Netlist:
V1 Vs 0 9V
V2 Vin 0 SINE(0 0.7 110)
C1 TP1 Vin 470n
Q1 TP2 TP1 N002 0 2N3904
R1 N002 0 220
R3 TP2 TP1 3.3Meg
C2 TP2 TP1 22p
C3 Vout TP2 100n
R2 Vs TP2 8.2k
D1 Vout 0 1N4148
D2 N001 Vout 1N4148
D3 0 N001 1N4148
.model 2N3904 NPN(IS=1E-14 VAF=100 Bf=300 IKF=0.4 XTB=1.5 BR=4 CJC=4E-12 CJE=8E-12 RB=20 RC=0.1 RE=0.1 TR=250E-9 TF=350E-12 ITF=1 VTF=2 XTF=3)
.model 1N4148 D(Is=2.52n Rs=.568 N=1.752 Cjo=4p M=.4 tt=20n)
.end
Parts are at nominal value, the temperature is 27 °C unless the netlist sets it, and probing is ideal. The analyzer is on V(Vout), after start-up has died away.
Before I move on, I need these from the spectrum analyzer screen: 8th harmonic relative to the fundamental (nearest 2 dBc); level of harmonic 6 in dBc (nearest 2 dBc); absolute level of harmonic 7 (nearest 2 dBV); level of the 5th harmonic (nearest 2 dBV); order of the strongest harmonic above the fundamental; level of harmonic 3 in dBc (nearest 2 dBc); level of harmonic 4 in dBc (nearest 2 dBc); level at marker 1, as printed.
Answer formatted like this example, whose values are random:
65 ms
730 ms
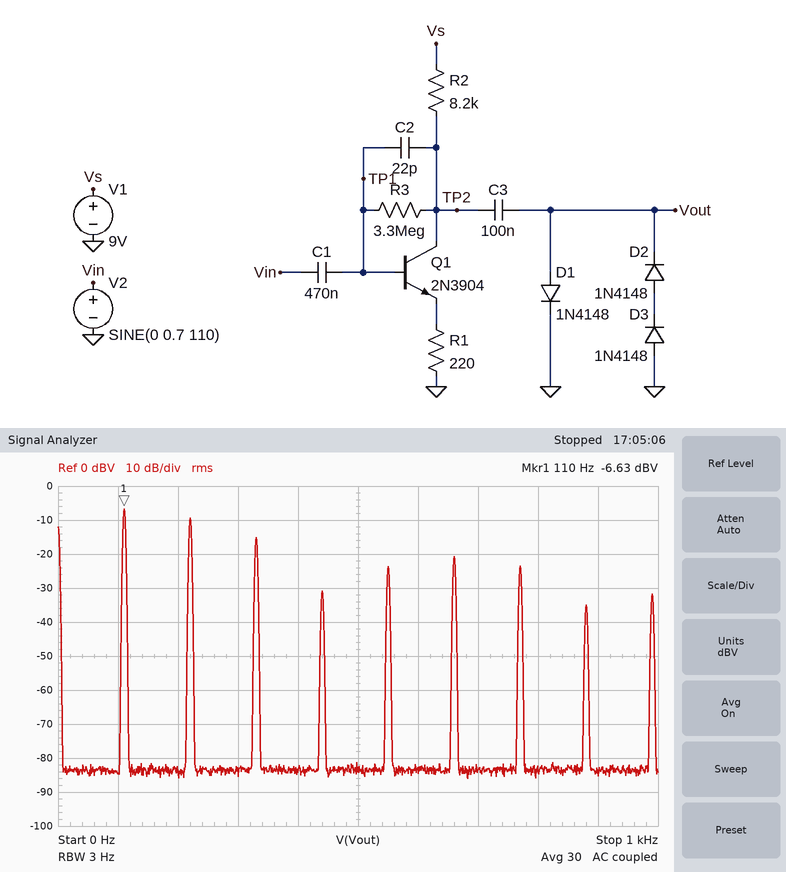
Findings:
-28 dBc
-14 dBc
-24 dBV
-24 dBV
2
-8 dBc
-24 dBc
-6.63 dBV
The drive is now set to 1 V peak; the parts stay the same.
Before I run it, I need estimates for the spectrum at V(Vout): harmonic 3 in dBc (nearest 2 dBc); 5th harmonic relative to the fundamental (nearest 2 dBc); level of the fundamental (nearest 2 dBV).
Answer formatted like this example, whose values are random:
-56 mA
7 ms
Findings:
-6 dBc
-32 dBc
-8 dBV
